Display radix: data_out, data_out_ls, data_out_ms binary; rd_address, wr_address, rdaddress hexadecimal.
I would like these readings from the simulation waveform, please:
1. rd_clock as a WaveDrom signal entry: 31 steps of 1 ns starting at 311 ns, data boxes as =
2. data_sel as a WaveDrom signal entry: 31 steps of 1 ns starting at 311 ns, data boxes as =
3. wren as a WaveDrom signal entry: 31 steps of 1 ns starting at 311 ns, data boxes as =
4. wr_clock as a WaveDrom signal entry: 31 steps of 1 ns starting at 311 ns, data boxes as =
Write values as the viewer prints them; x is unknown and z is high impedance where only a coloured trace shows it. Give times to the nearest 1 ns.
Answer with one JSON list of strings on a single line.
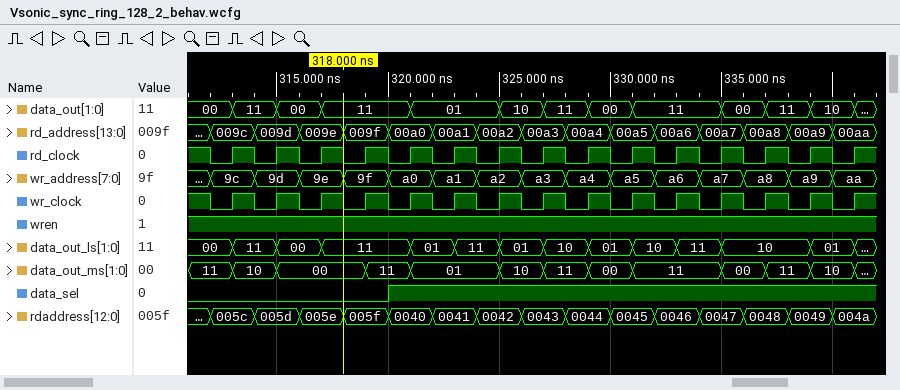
["{name: 'rd_clock', wave: '1010101010101010101010101010101'}", "{name: 'data_sel', wave: '0........1.....................'}", "{name: 'wren', wave: '1..............................'}", "{name: 'wr_clock', wave: '1010101010101010101010101010101'}"]
